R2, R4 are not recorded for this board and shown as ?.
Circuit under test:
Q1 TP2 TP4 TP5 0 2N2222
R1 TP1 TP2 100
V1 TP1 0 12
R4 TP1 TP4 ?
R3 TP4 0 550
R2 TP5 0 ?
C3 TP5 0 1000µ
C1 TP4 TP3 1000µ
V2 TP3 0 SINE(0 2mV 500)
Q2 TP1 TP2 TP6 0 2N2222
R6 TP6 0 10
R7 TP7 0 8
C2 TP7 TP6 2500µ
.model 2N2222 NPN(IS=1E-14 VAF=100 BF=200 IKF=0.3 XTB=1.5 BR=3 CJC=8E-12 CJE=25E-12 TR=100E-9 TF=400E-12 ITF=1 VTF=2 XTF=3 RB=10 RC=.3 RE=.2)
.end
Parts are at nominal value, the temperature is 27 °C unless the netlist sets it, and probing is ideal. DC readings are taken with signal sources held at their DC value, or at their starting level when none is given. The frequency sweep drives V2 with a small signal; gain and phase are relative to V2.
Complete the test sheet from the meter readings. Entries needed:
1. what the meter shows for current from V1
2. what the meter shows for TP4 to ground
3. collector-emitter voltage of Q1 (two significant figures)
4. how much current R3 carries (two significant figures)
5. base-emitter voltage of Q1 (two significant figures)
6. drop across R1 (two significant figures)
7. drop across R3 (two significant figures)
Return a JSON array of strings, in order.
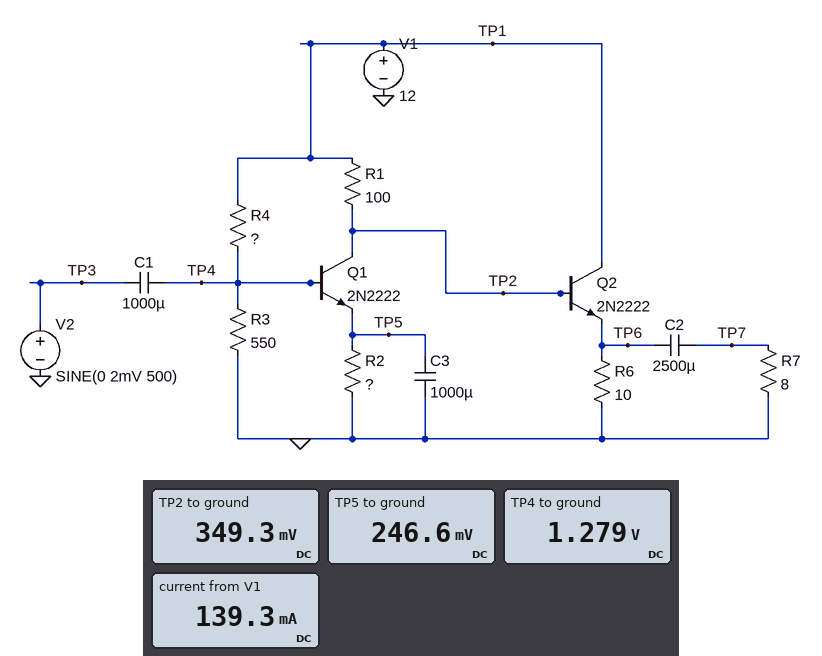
["139.3 mA", "1.279 V", "100 mV", "2.3 mA", "1.0 V", "12 V", "1.3 V"]
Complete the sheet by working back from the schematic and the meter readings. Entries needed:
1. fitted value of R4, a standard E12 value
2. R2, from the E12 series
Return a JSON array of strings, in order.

["470 Ω", "1.8 Ω"]
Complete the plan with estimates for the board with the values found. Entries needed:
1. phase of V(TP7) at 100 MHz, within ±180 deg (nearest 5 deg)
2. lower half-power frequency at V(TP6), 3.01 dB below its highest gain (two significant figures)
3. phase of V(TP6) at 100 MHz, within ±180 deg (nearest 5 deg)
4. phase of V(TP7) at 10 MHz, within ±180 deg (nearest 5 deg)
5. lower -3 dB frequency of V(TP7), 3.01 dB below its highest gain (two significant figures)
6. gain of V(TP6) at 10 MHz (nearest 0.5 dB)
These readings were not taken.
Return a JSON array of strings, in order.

["65 deg", "160 MHz", "65 deg", "95 deg", "160 MHz", "-70.0 dB"]
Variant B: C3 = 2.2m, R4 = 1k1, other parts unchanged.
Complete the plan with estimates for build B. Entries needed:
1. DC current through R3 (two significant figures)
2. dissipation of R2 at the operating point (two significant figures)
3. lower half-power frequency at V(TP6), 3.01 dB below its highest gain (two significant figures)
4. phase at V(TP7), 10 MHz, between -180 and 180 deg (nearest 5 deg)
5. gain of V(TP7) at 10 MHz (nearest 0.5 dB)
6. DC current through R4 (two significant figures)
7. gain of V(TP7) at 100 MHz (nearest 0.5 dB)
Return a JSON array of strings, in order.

["2.0 mA", "28 mW", "150 MHz", "110 deg", "-68.5 dB", "9.9 mA", "-49.5 dB"]
